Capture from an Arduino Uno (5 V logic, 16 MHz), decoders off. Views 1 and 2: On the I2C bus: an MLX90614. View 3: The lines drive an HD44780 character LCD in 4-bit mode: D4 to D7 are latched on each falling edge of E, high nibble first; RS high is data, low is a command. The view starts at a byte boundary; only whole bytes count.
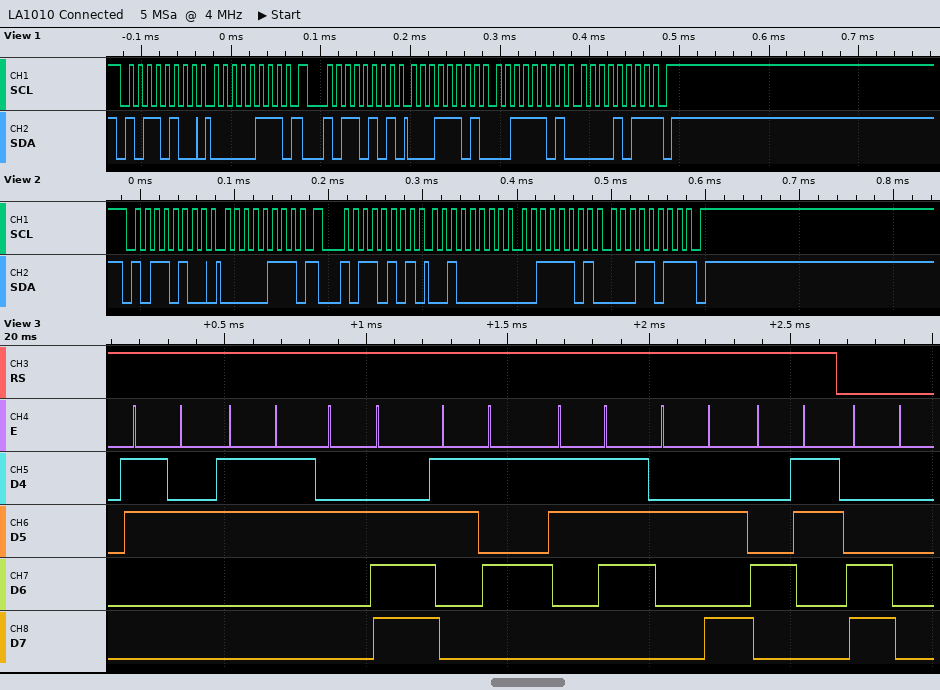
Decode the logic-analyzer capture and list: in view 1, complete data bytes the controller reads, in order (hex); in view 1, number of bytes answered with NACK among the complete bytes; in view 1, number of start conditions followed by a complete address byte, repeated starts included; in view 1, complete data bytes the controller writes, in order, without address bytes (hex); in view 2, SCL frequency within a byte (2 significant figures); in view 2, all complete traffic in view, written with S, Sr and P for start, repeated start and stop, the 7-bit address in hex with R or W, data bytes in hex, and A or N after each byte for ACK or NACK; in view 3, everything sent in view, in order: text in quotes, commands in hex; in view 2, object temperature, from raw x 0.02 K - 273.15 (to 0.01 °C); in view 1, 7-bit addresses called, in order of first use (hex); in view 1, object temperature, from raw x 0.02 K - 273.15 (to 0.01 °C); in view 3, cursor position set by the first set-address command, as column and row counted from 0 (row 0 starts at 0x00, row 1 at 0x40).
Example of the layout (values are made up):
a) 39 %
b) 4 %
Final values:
a) 1D 3D 0B
b) 1
c) 2
d) 07
e) 100 kHz
f) S 5AW A 07 A Sr 5AR A 20 A 3D A 1B N P
g) "23.57*C" 0xC0
h) 39.81 °C
i) 0x5A
j) 39.75 °C
k) column 0, row 1
